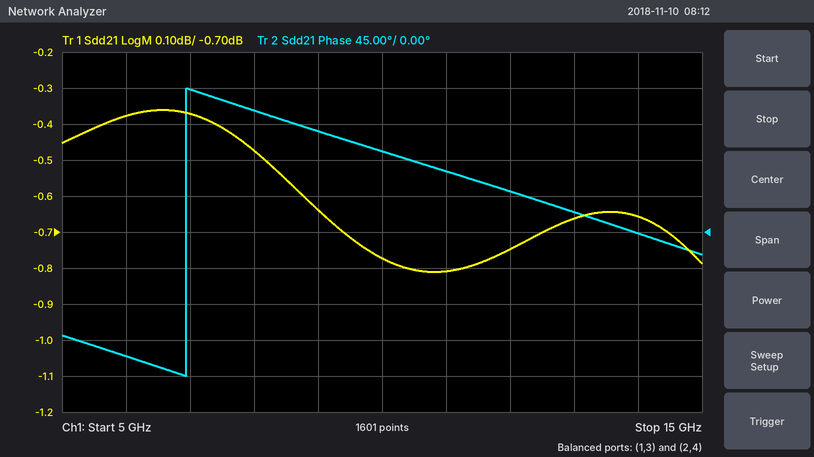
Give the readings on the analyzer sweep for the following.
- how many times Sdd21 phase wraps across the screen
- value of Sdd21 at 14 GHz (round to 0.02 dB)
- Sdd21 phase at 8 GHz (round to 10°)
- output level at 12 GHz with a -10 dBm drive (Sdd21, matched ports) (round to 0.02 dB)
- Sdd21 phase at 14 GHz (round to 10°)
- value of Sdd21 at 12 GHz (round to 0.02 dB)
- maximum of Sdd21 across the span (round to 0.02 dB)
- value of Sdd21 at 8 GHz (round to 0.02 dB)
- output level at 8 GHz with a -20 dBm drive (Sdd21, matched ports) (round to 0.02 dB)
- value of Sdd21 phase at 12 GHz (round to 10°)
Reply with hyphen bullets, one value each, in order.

- 1
- -0.66 dB
- 150°
- -10.74 dBm
- 0°
- -0.74 dB
- -0.36 dB
- -0.48 dB
- -20.48 dBm
- 50°
